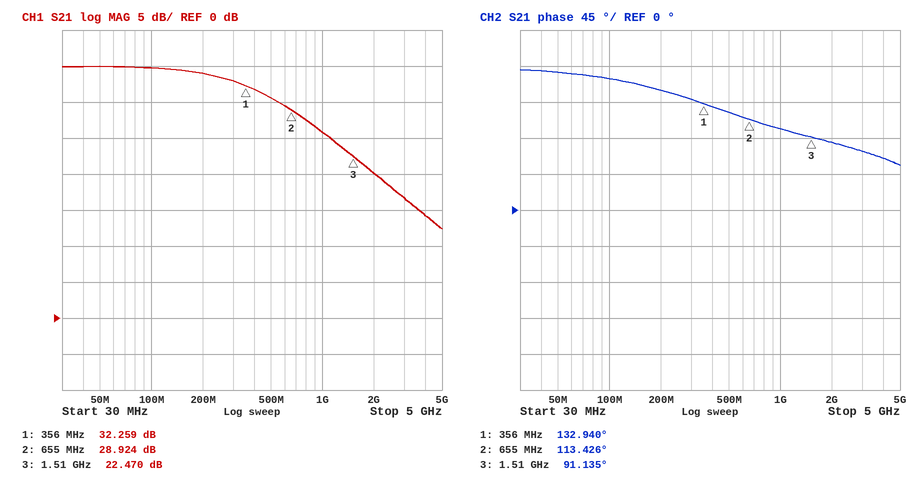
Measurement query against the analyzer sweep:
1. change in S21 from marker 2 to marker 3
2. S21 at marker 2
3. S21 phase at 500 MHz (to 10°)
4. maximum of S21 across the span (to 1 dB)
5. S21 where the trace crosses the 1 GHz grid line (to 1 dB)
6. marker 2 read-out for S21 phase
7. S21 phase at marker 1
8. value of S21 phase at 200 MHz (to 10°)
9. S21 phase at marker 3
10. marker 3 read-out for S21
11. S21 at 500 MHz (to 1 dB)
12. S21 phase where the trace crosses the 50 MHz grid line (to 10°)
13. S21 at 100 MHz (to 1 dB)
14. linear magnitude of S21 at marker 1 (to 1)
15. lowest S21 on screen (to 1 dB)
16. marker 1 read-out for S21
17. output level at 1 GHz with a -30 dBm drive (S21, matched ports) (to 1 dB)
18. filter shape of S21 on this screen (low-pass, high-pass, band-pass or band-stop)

-6.454 dB
28.924 dB
120°
35 dB
26 dB
113.426°
132.940°
150°
91.135°
22.470 dB
31 dB
170°
35 dB
41
12 dB
32.259 dB
-4 dBm
low-pass
